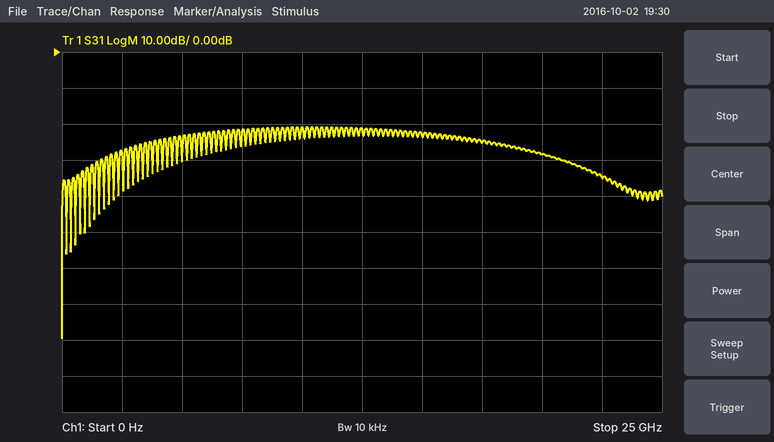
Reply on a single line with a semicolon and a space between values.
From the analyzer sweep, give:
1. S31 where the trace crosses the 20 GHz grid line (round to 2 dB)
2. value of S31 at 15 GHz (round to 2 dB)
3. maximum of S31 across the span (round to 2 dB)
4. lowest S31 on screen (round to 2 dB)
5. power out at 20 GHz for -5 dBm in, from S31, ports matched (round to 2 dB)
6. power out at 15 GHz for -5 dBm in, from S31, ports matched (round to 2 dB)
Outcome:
-28 dB; -24 dB; -20 dB; -80 dB; -34 dBm; -28 dBm
